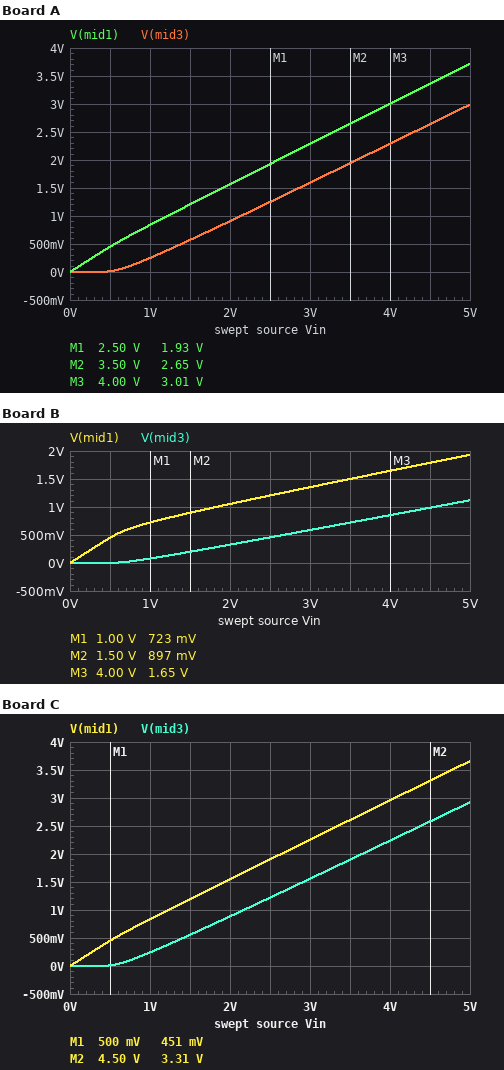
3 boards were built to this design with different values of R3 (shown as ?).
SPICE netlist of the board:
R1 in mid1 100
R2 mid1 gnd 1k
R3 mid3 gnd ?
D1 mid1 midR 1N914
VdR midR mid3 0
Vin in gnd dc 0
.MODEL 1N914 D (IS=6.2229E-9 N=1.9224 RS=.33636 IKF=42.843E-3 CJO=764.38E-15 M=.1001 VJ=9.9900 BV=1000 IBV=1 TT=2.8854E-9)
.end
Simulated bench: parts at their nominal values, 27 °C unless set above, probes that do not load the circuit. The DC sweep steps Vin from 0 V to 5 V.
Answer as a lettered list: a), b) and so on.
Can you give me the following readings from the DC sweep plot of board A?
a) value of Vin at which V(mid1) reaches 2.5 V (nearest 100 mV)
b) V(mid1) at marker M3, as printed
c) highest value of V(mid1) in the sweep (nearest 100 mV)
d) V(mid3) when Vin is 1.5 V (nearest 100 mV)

a) 3.3 V
b) 3.01 V
c) 3.7 V
d) 600 mV
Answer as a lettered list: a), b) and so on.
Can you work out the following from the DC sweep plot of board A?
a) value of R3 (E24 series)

a) 330 Ω
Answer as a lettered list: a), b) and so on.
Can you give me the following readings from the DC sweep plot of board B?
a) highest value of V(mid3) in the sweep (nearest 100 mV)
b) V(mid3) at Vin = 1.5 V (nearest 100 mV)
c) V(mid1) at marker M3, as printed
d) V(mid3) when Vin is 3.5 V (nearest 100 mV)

a) 1.1 V
b) 200 mV
c) 1.65 V
d) 700 mV
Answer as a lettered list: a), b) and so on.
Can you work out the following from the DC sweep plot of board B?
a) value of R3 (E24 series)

a) 39 Ω
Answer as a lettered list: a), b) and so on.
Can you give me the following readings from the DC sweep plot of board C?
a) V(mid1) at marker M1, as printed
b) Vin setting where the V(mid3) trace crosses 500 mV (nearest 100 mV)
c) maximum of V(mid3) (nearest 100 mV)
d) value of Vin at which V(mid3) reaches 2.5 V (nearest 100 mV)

a) 451 mV
b) 1.4 V
c) 2.9 V
d) 4.4 V
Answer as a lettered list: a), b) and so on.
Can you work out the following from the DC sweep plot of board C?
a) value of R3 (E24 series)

a) 300 Ω
